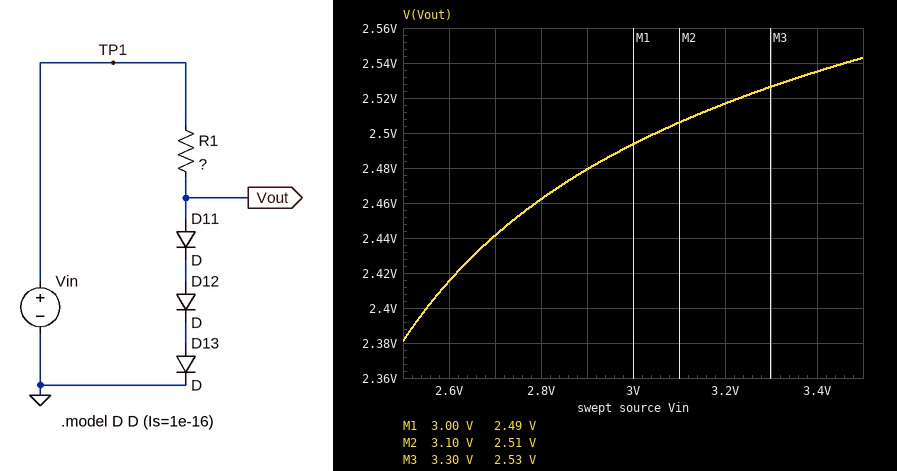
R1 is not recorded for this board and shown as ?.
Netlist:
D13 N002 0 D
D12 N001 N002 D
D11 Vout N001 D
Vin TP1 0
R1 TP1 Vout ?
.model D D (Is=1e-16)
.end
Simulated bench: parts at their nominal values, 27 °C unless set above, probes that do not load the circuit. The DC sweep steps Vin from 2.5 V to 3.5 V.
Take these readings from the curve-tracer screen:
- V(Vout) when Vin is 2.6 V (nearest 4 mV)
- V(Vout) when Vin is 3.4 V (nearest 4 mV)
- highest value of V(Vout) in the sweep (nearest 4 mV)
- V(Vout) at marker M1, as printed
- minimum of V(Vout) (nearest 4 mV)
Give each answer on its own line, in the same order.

2.416 V
2.536 V
2.544 V
2.49 V
2.380 V
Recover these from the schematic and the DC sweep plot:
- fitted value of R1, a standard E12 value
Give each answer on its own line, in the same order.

56 Ω
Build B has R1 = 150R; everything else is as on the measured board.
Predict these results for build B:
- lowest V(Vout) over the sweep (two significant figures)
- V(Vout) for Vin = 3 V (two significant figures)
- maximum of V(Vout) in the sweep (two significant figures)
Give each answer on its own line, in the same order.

2.3 V
2.4 V
2.5 V
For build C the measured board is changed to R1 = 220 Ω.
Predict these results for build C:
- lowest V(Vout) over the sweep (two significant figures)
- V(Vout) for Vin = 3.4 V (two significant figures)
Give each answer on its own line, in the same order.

2.3 V
2.4 V
